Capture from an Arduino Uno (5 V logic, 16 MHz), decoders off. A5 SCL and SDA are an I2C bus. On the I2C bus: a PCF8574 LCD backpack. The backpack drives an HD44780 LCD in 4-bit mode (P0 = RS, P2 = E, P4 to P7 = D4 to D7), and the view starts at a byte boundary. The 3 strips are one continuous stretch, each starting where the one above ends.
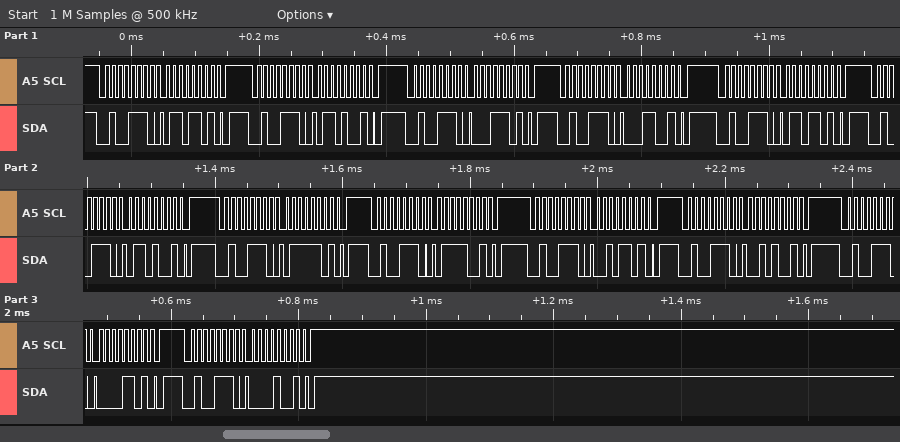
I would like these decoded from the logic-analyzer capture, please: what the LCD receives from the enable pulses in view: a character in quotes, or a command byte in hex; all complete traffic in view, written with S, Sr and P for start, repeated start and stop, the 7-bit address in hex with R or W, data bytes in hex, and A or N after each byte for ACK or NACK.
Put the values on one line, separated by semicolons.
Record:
'a' 'g' ' '; S 27W A 6D A P S 27W A 69 A P S 27W A 1D A P S 27W A 19 A P S 27W A 6D A P S 27W A 69 A P S 27W A 7D A P S 27W A 79 A P S 27W A 2D A P S 27W A 29 A P S 27W A 0D A P S 27W A 09 A P
